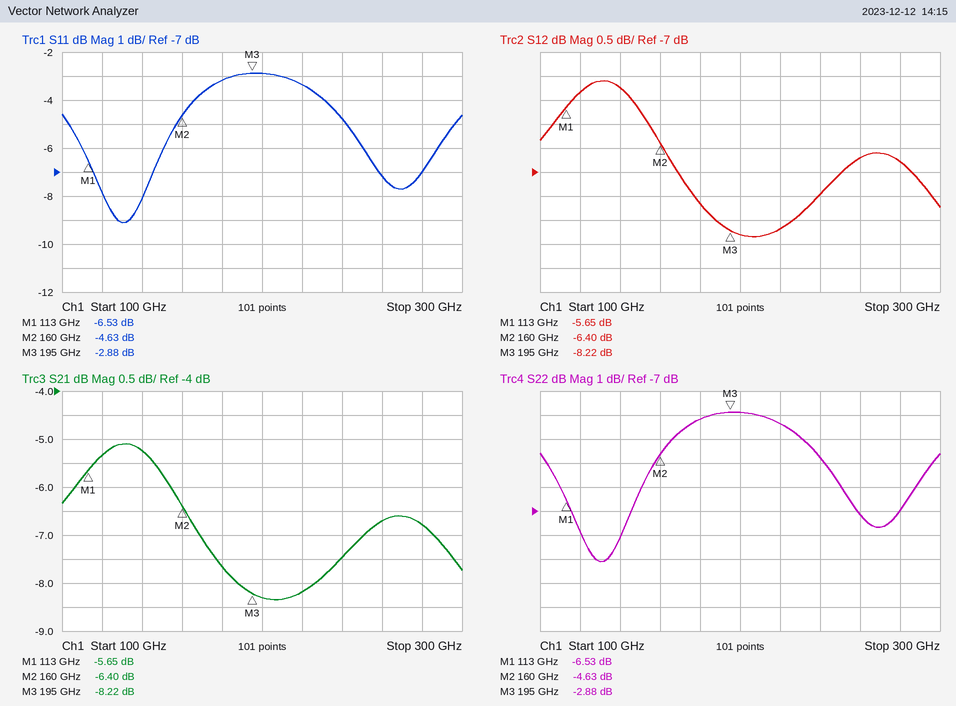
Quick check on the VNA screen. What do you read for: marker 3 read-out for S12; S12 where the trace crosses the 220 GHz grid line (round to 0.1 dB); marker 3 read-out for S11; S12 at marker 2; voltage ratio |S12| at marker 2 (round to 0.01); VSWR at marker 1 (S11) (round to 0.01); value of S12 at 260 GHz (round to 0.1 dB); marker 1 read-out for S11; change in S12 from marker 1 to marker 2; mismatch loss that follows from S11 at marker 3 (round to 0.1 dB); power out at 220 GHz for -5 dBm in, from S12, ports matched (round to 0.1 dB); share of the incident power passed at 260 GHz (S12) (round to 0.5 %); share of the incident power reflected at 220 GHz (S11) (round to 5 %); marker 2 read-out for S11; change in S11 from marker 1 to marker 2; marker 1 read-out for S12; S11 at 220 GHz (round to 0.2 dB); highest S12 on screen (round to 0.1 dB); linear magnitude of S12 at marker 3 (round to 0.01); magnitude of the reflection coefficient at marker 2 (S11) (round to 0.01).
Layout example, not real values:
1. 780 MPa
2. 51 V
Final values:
1. -8.22 dB
2. -8.2 dB
3. -2.88 dB
4. -6.40 dB
5. 0.48
6. 2.78
7. -6.7 dB
8. -6.53 dB
9. -0.75 dB
10. 3.1 dB
11. -13.2 dBm
12. 21.5 %
13. 45 %
14. -4.63 dB
15. 1.90 dB
16. -5.65 dB
17. -3.4 dB
18. -5.1 dB
19. 0.39
20. 0.59
